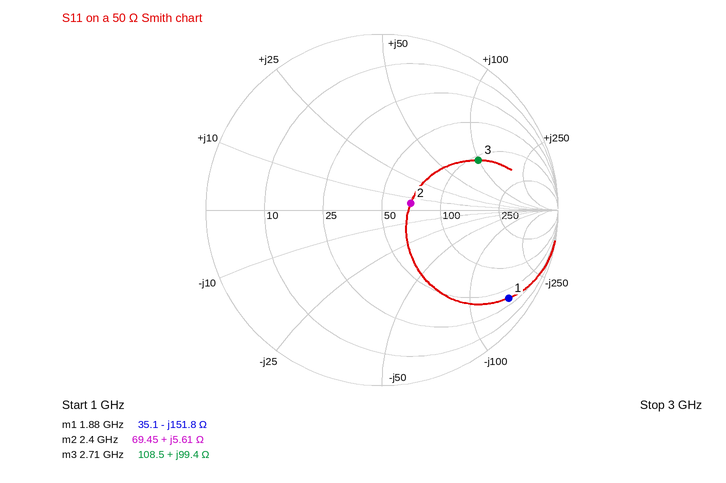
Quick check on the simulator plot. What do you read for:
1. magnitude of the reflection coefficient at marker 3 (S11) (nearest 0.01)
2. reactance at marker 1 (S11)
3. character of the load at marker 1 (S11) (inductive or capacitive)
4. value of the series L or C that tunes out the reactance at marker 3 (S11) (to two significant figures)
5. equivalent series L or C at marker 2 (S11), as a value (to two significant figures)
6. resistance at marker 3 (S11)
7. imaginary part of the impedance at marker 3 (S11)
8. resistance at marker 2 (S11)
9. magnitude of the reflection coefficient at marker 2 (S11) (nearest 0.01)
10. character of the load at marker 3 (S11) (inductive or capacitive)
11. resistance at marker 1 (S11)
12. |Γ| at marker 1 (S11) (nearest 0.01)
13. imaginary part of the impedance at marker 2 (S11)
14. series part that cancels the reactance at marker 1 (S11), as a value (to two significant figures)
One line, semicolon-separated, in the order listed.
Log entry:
0.62; -151.8 Ω; capacitive; 590 fF; 370 pH; 108.5 Ω; +99.4 Ω; 69.45 Ω; 0.17; inductive; 35.1 Ω; 0.88; +5.61 Ω; 13 nH
